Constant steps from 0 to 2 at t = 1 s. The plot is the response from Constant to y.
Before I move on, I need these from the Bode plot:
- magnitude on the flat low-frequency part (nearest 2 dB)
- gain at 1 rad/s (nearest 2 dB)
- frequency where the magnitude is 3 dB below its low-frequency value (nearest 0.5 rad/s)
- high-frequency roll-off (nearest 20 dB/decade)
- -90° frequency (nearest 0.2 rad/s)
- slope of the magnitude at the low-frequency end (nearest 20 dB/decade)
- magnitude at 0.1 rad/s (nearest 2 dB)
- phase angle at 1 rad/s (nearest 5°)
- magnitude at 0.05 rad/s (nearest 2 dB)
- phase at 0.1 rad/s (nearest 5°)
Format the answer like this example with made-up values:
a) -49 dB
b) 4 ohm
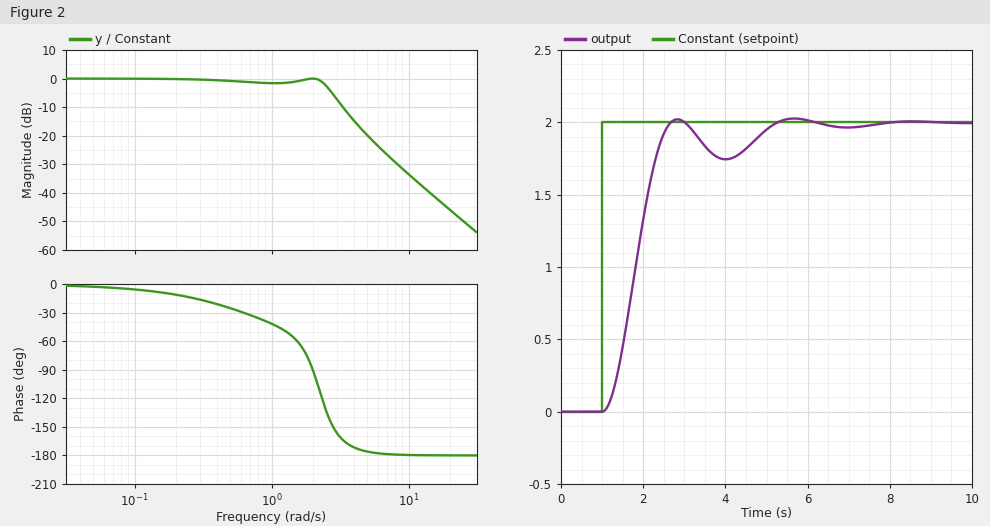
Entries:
a) 0 dB
b) -2 dB
c) 2.5 rad/s
d) -40 dB/decade
e) 2.0 rad/s
f) 0 dB/decade
g) 0 dB
h) -40°
i) 0 dB
j) -5°
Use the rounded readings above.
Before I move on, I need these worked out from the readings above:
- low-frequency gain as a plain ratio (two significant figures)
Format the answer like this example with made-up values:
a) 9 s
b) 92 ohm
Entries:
a) 1.0
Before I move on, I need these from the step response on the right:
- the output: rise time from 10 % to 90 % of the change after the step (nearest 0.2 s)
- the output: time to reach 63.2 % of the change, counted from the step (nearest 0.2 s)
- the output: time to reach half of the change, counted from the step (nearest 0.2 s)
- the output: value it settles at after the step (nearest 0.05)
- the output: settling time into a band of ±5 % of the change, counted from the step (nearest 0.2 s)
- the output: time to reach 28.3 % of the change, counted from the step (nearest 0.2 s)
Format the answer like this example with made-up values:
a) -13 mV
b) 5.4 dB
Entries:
a) 1.0 s
b) 1.0 s
c) 0.8 s
d) 2.00
e) 3.8 s
f) 0.6 s
